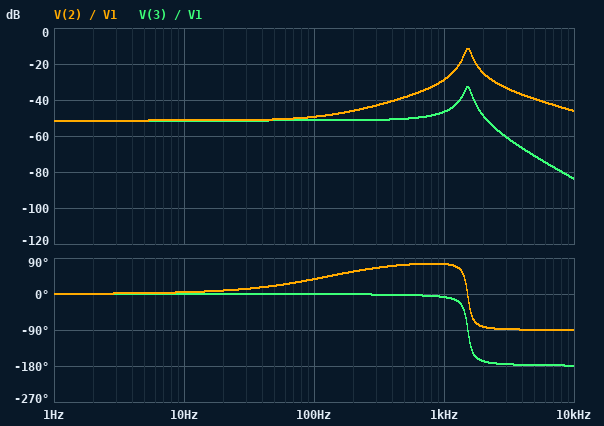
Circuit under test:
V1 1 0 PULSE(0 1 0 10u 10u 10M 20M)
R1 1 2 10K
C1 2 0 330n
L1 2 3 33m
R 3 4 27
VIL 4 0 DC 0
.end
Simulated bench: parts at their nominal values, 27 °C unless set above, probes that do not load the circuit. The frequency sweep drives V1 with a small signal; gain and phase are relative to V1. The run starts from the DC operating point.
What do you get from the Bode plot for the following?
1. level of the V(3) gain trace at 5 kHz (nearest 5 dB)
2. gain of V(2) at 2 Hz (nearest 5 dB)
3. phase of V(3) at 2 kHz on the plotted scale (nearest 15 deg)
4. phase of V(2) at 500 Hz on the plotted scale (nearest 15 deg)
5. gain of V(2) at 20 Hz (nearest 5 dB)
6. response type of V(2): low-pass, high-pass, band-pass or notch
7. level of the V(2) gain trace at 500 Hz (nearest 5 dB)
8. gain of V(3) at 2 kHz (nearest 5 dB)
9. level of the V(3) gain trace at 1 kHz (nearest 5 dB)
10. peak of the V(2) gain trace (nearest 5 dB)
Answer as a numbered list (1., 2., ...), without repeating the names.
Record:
1. -70 dB
2. -50 dB
3. -165 deg
4. 75 deg
5. -50 dB
6. band-pass
7. -40 dB
8. -50 dB
9. -45 dB
10. -10 dB
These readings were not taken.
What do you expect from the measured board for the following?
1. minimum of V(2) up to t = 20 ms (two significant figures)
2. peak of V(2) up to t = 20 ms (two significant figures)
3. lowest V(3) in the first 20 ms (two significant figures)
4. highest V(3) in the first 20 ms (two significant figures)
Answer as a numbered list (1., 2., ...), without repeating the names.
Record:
1. -29 mV
2. 31 mV
3. -2.2 mV
4. 4.9 mV
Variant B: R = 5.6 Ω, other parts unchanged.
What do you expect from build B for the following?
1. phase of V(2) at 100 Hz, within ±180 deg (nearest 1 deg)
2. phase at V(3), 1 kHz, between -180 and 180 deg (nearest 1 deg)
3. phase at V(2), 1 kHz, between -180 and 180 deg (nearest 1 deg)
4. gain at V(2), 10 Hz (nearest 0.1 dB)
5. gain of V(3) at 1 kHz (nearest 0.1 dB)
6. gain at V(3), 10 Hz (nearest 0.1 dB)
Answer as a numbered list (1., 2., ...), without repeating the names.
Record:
1. 75 deg
2. -3 deg
3. 85 deg
4. -64.5 dB
5. -60.2 dB
6. -65.0 dB
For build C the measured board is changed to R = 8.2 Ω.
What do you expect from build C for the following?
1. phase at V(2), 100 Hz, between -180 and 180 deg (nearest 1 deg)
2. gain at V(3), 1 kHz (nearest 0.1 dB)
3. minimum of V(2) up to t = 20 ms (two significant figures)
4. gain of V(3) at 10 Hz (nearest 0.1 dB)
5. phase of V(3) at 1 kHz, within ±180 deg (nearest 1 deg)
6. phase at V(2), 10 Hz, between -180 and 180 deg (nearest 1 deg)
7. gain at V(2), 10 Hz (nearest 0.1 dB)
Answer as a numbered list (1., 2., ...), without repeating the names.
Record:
1. 68 deg
2. -56.9 dB
3. -30 mV
4. -61.7 dB
5. -4 deg
6. 14 deg
7. -61.5 dB
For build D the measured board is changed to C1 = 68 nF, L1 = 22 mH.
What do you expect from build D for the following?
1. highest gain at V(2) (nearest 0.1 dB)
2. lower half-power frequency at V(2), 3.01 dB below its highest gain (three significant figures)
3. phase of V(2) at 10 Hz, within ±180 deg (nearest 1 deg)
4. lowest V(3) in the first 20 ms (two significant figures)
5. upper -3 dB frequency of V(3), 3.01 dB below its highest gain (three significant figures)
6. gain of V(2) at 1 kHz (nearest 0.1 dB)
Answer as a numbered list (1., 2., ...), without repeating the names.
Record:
1. -5.3 dB
2. 3.91 kHz
3. 3 deg
4. -2.3 mV
5. 4.32 kHz
6. -36.5 dB
